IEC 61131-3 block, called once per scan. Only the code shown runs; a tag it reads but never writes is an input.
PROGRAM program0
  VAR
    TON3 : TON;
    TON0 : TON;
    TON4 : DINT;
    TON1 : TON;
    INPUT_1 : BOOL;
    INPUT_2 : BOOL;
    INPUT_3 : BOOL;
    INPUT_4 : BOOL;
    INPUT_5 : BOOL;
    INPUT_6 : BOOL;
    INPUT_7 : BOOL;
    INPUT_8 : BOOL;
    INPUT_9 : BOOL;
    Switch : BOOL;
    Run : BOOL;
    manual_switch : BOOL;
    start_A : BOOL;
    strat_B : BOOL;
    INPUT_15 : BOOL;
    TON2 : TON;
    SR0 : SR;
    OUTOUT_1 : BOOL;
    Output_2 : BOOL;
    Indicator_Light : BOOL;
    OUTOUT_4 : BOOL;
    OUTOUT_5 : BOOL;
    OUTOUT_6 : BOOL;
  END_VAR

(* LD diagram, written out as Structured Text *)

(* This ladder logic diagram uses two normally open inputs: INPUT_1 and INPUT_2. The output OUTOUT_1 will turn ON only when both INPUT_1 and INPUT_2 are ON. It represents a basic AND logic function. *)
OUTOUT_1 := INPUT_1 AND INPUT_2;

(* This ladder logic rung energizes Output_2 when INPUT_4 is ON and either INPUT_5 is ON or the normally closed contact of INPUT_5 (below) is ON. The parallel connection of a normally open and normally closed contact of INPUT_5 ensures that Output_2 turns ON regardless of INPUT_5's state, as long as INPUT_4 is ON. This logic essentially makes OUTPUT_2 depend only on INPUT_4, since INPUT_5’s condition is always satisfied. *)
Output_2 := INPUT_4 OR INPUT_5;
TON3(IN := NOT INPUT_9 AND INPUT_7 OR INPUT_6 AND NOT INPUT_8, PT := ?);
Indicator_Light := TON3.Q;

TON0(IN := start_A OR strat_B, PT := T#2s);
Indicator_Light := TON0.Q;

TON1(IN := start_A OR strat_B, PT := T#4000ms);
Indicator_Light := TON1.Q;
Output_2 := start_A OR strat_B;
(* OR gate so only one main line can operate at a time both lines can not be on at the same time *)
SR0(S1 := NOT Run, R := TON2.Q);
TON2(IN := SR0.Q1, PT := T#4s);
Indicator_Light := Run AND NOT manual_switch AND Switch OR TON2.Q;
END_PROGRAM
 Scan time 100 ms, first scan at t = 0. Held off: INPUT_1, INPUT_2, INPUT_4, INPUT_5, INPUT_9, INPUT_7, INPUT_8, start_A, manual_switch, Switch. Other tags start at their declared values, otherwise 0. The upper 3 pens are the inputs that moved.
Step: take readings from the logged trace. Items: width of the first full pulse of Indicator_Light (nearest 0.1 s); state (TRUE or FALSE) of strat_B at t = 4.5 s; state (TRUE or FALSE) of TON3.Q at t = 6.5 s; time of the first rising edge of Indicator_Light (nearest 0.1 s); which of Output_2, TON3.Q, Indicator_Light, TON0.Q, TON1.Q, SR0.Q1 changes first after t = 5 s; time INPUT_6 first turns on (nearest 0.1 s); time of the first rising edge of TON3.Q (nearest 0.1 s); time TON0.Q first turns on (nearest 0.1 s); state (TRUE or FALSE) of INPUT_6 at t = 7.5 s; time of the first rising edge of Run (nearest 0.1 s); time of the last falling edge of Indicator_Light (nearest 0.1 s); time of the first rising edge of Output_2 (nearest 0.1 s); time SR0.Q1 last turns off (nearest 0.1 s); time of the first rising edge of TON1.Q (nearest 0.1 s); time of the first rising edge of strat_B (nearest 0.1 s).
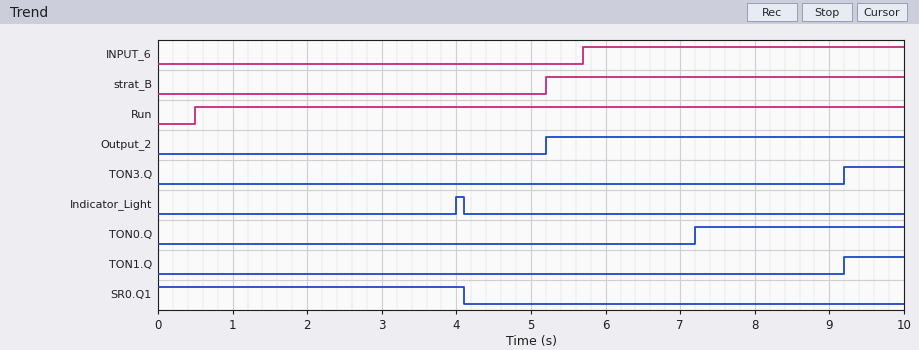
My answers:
0.1 s
FALSE
FALSE
4.0 s
Output_2
5.7 s
9.2 s
7.2 s
TRUE
0.5 s
4.1 s
5.2 s
4.1 s
9.2 s
5.2 s
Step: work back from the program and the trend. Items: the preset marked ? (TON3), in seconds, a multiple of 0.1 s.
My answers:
3.5 s
